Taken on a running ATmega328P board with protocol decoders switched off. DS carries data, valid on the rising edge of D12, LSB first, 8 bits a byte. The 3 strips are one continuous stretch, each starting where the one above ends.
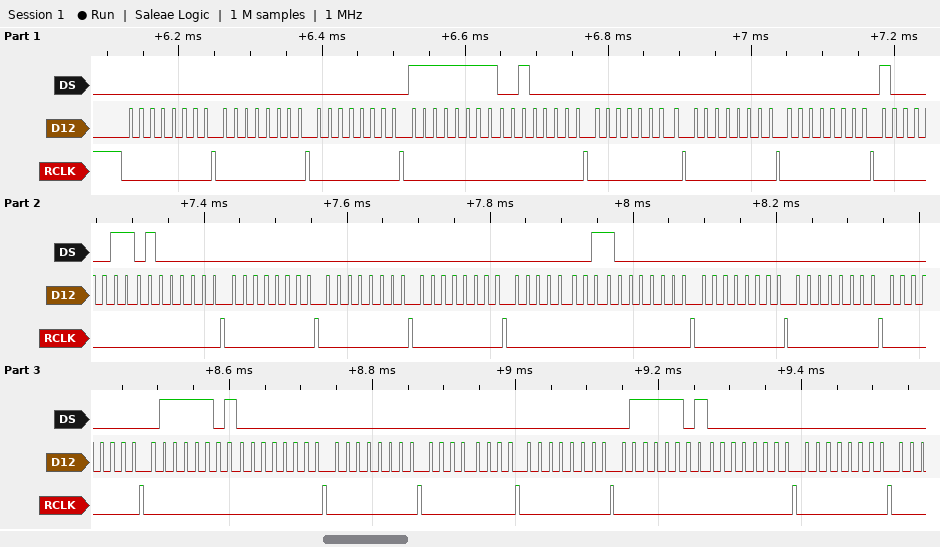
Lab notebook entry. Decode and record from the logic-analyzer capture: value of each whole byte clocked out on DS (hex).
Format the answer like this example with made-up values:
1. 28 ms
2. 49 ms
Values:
1. 00 00 00 FF 04 00 00 00 C1 02 00 00 00 80 01 00 00 00 BE 00 00 00 00 BE 00 00
